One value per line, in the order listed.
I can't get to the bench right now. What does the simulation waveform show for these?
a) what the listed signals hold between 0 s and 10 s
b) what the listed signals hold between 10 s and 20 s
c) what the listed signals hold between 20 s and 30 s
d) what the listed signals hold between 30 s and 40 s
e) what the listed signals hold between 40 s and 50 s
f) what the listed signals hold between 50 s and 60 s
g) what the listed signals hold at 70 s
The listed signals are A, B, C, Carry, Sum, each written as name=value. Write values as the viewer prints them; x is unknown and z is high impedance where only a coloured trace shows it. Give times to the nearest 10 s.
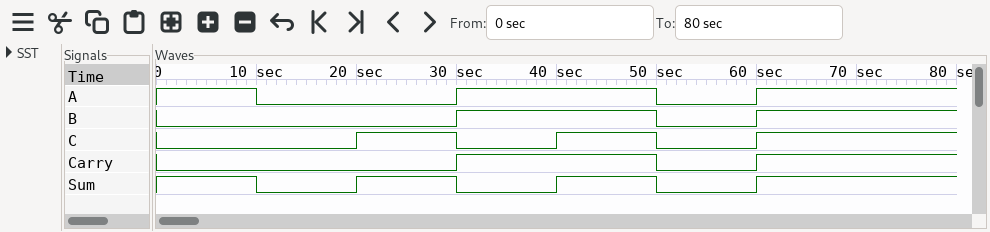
A=1, B=0, C=0, Carry=0, Sum=1
A=0, B=0, C=0, Carry=0, Sum=0
A=0, B=0, C=1, Carry=0, Sum=1
A=1, B=1, C=0, Carry=1, Sum=0
A=1, B=1, C=1, Carry=1, Sum=1
A=0, B=0, C=0, Carry=0, Sum=0
A=1, B=1, C=1, Carry=1, Sum=1
